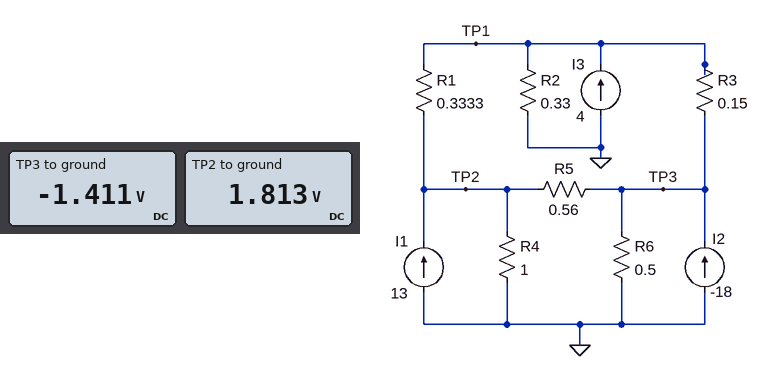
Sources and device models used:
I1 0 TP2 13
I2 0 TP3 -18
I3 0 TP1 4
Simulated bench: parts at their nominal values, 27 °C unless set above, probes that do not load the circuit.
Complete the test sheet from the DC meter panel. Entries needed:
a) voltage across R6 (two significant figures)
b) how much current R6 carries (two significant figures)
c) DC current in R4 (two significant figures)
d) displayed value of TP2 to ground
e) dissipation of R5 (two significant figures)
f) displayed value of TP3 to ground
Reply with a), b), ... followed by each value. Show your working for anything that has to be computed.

a) 0 V - (-1.411 V) = 1.4 V
b) (0 V - (-1.411 V)) / 500 mΩ = 2.8 A
c) (1.813 V) / 1 Ω = 1.8 A
d) 1.813 V
e) (1.813 V - (-1.411 V))^2 / 560 mΩ = 19 W
f) -1.411 V
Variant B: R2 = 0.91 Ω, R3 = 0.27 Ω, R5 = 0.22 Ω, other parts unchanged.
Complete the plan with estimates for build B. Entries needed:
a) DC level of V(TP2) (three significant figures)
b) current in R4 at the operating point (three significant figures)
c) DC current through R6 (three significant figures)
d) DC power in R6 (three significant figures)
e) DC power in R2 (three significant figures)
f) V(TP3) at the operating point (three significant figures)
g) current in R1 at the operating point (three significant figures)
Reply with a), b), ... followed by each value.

a) 1.01 V
b) 1.01 A
c) 2.38 A
d) 2.82 W
e) 124 mW
f) -1.19 V
g) 2.01 A
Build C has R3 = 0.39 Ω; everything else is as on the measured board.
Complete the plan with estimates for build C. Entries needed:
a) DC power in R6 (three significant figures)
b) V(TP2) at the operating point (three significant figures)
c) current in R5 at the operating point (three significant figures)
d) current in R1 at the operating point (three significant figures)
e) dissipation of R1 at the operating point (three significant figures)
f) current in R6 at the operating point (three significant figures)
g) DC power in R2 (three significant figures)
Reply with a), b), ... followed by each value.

a) 9.07 W
b) 1.83 V
c) 7.08 A
d) 4.09 A
e) 5.58 W
f) 4.26 A
g) 670 mW
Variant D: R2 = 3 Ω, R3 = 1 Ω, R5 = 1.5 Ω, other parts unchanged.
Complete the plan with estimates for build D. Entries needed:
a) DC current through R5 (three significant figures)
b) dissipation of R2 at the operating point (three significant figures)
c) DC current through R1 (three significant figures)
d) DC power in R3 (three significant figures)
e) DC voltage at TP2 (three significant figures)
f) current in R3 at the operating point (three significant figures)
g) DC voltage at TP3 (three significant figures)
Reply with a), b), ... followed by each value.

a) 5.08 A
b) 3.45 W
c) 3.52 A
d) 41.6 W
e) 4.39 V
f) 6.45 A
g) -3.23 V
